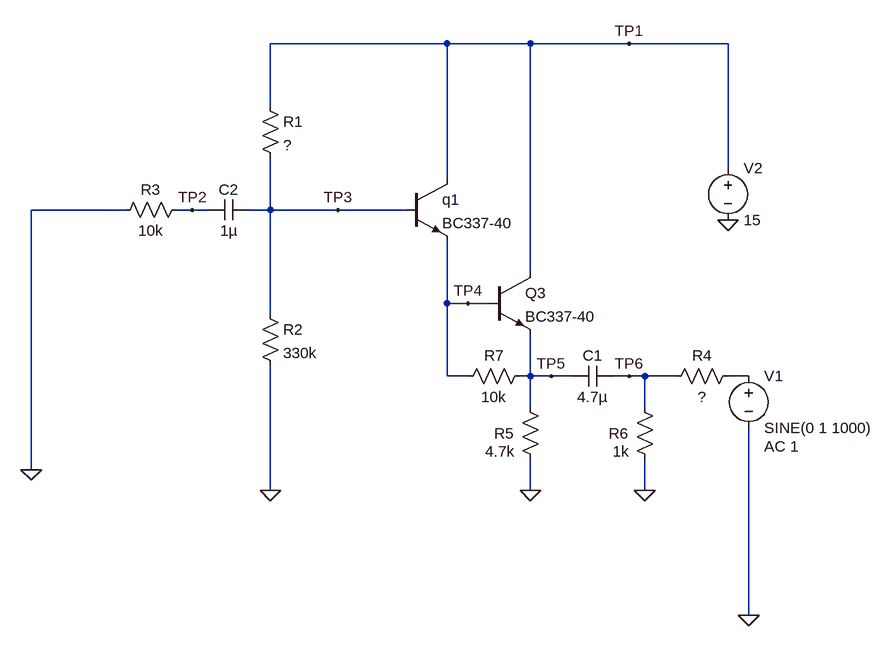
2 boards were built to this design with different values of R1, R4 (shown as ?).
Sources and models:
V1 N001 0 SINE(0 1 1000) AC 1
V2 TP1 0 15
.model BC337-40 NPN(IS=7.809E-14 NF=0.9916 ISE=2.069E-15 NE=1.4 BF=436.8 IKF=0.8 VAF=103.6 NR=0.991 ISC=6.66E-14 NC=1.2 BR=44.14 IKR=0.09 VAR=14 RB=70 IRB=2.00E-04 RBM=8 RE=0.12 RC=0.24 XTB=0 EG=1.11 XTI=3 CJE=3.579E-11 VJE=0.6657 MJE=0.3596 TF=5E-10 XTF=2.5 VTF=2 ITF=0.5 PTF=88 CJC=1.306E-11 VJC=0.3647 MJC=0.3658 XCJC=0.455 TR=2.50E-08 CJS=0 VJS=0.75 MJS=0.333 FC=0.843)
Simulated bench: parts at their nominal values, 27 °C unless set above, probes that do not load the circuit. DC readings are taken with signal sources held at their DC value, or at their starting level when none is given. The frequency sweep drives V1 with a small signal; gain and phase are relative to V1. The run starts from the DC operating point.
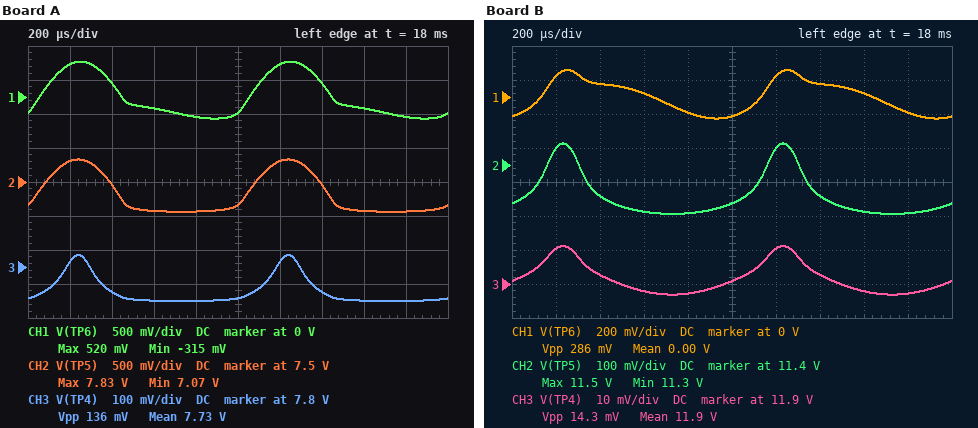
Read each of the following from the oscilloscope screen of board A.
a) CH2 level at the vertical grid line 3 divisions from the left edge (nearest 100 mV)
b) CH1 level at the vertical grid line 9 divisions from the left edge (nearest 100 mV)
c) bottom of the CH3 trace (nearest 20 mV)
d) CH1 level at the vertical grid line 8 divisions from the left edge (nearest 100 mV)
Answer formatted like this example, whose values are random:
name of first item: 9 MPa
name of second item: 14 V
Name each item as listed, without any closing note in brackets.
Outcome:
CH2 level at the vertical grid line 3 divisions from the left edge: 7.1 V
CH1 level at the vertical grid line 9 divisions from the left edge: -300 mV
bottom of the CH3 trace: 7.70 V
CH1 level at the vertical grid line 8 divisions from the left edge: -200 mV
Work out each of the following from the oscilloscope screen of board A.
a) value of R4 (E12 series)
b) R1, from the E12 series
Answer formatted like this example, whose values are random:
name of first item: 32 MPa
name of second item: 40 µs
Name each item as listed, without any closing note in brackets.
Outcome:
value of R4: 220 Ω
R1, from the E12 series: 270 kΩ
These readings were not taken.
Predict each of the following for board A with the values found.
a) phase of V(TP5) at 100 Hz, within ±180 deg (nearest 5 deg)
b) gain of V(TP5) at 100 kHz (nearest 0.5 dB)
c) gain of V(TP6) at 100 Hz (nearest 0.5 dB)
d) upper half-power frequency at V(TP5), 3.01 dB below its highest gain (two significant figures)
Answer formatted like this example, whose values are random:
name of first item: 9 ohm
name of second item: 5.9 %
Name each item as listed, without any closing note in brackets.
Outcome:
phase of V(TP5) at 100 Hz, within ±180 deg: 60 deg
gain of V(TP5) at 100 kHz: -22.0 dB
gain of V(TP6) at 100 Hz: -3.0 dB
upper half-power frequency at V(TP5), 3.01 dB below its highest gain: 350 MHz
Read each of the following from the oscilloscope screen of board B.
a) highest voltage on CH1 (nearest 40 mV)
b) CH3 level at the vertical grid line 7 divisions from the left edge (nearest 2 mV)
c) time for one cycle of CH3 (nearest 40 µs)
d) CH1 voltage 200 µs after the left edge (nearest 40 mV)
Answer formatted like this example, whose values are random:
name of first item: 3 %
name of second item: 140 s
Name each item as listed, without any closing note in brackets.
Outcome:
highest voltage on CH1: 160 mV
CH3 level at the vertical grid line 7 divisions from the left edge: 11.902 V
time for one cycle of CH3: 1.00 ms
CH1 voltage 200 µs after the left edge: 120 mV
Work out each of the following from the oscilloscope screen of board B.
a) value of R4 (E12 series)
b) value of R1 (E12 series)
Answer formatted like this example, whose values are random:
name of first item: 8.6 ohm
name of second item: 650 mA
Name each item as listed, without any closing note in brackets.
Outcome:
value of R4: 330 Ω
value of R1: 68 kΩ
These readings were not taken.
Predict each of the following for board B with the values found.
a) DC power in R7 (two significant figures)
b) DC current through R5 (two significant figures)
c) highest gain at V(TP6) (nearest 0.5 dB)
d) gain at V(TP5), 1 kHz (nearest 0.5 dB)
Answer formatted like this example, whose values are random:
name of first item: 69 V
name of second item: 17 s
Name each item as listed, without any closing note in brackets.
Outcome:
DC power in R7: 38 µW
DC current through R5: 2.4 mA
highest gain at V(TP6): -2.5 dB
gain at V(TP5), 1 kHz: -29.0 dB
